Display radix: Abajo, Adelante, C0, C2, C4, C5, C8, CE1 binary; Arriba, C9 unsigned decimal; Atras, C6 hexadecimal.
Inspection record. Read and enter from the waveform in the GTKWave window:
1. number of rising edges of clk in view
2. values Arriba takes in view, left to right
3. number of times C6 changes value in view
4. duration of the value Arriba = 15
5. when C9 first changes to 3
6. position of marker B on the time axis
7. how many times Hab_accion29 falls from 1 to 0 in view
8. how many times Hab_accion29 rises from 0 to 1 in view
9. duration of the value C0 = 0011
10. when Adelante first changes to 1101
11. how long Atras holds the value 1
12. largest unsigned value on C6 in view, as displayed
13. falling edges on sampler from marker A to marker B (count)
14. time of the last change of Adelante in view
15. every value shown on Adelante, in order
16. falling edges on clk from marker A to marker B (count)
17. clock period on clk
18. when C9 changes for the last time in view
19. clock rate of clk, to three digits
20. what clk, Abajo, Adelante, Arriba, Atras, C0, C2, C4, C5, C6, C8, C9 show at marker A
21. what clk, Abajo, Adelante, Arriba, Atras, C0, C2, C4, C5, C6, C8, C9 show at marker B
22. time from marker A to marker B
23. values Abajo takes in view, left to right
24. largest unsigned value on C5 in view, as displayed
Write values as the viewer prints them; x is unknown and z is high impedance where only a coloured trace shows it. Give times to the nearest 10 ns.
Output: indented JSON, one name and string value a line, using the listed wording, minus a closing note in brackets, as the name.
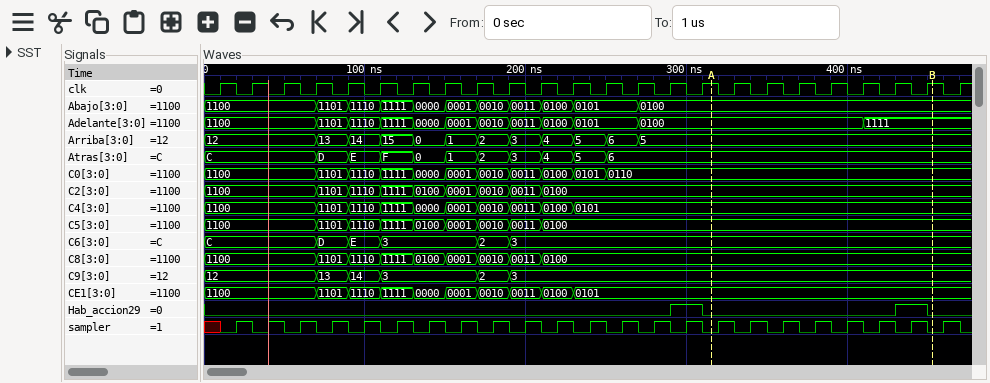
{
  "number of rising edges of clk in view": "24",
  "values Arriba takes in view, left to right": "12, 13, 14, 15, 0, 1, 2, 3, 4, 5, 6, 5",
  "number of times C6 changes value in view": "5",
  "duration of the value Arriba = 15": "20 ns",
  "when C9 first changes to 3": "110 ns",
  "position of marker B on the time axis": "450 ns",
  "how many times Hab_accion29 falls from 1 to 0 in view": "2",
  "how many times Hab_accion29 rises from 0 to 1 in view": "2",
  "duration of the value C0 = 0011": "20 ns",
  "when Adelante first changes to 1101": "70 ns",
  "how long Atras holds the value 1": "20 ns",
  "largest unsigned value on C6 in view, as displayed": "E",
  "falling edges on sampler from marker A to marker B": "7",
  "time of the last change of Adelante in view": "410 ns",
  "every value shown on Adelante, in order": "1100, 1101, 1110, 1111, 0000, 0001, 0010, 0011, 0100, 0101, 0100, 1111",
  "falling edges on clk from marker A to marker B": "7",
  "clock period on clk": "20 ns",
  "when C9 changes for the last time in view": "190 ns",
  "clock rate of clk, to three digits": "50.0 MHz",
  "what clk, Abajo, Adelante, Arriba, Atras, C0, C2, C4, C5, C6, C8, C9 show at marker A": "clk=1, Abajo=0100, Adelante=0100, Arriba=5, Atras=6, C0=0110, C2=0100, C4=0101, C5=0100, C6=3, C8=0100, C9=3",
  "what clk, Abajo, Adelante, Arriba, Atras, C0, C2, C4, C5, C6, C8, C9 show at marker B": "clk=1, Abajo=0100, Adelante=1111, Arriba=5, Atras=6, C0=0110, C2=0100, C4=0101, C5=0100, C6=3, C8=0100, C9=3",
  "time from marker A to marker B": "140 ns",
  "values Abajo takes in view, left to right": "1100, 1101, 1110, 1111, 0000, 0001, 0010, 0011, 0100, 0101, 0100",
  "largest unsigned value on C5 in view, as displayed": "1111"
}
